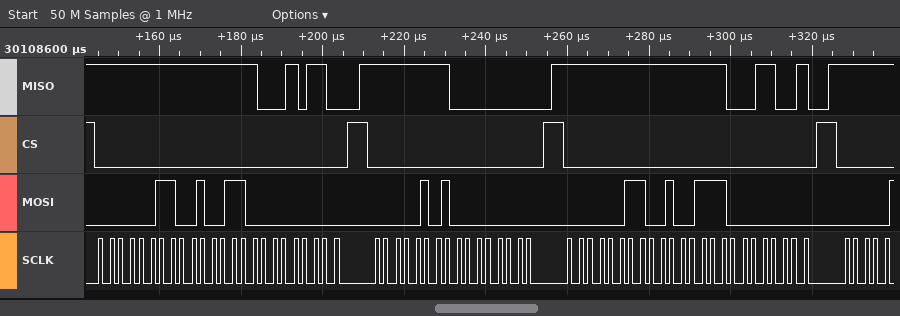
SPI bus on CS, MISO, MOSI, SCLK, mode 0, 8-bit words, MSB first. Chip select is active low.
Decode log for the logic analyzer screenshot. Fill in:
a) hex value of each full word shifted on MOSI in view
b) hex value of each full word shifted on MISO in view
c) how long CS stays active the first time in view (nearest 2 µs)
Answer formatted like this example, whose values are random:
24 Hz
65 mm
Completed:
03, 26, 00, 05, 00, 03, 27, 00
FF, FF, 16, FF, 00, FF, FF, 19
62 µs
